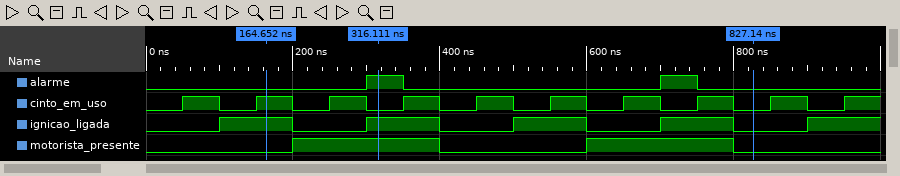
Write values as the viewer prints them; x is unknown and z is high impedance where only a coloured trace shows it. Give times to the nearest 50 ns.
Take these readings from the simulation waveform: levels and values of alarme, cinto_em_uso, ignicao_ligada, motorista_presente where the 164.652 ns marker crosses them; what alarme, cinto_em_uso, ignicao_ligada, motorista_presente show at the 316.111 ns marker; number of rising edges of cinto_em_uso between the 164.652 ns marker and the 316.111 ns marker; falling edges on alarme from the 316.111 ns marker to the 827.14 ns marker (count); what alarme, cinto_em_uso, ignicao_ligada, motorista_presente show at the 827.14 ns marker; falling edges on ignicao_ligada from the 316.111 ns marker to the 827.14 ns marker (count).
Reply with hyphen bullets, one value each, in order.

- alarme=0, cinto_em_uso=1, ignicao_ligada=1, motorista_presente=0
- alarme=1, cinto_em_uso=0, ignicao_ligada=1, motorista_presente=1
- 1
- 2
- alarme=0, cinto_em_uso=0, ignicao_ligada=0, motorista_presente=0
- 3
